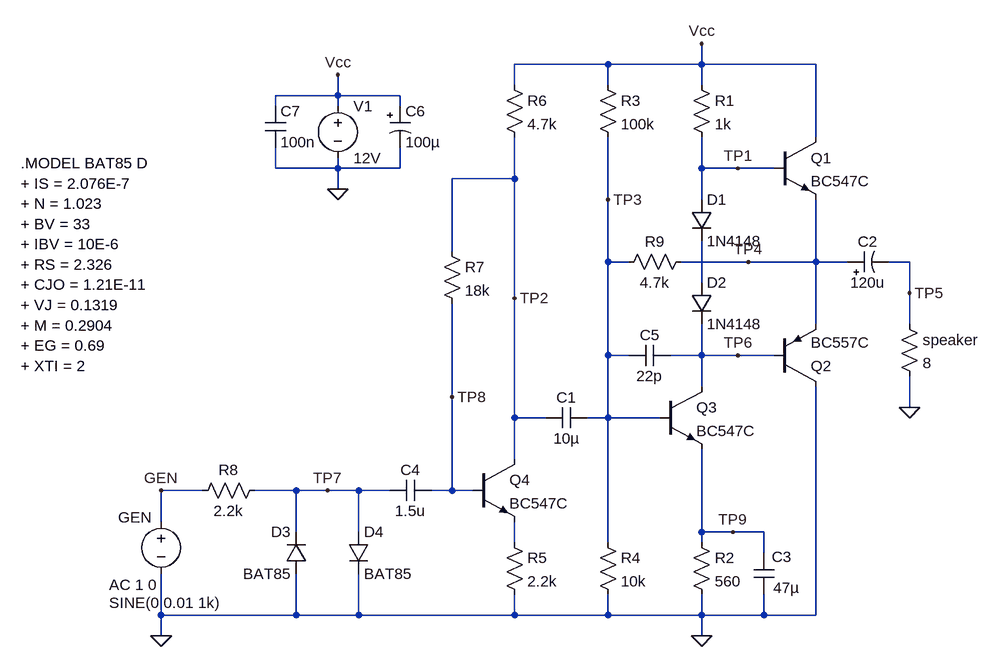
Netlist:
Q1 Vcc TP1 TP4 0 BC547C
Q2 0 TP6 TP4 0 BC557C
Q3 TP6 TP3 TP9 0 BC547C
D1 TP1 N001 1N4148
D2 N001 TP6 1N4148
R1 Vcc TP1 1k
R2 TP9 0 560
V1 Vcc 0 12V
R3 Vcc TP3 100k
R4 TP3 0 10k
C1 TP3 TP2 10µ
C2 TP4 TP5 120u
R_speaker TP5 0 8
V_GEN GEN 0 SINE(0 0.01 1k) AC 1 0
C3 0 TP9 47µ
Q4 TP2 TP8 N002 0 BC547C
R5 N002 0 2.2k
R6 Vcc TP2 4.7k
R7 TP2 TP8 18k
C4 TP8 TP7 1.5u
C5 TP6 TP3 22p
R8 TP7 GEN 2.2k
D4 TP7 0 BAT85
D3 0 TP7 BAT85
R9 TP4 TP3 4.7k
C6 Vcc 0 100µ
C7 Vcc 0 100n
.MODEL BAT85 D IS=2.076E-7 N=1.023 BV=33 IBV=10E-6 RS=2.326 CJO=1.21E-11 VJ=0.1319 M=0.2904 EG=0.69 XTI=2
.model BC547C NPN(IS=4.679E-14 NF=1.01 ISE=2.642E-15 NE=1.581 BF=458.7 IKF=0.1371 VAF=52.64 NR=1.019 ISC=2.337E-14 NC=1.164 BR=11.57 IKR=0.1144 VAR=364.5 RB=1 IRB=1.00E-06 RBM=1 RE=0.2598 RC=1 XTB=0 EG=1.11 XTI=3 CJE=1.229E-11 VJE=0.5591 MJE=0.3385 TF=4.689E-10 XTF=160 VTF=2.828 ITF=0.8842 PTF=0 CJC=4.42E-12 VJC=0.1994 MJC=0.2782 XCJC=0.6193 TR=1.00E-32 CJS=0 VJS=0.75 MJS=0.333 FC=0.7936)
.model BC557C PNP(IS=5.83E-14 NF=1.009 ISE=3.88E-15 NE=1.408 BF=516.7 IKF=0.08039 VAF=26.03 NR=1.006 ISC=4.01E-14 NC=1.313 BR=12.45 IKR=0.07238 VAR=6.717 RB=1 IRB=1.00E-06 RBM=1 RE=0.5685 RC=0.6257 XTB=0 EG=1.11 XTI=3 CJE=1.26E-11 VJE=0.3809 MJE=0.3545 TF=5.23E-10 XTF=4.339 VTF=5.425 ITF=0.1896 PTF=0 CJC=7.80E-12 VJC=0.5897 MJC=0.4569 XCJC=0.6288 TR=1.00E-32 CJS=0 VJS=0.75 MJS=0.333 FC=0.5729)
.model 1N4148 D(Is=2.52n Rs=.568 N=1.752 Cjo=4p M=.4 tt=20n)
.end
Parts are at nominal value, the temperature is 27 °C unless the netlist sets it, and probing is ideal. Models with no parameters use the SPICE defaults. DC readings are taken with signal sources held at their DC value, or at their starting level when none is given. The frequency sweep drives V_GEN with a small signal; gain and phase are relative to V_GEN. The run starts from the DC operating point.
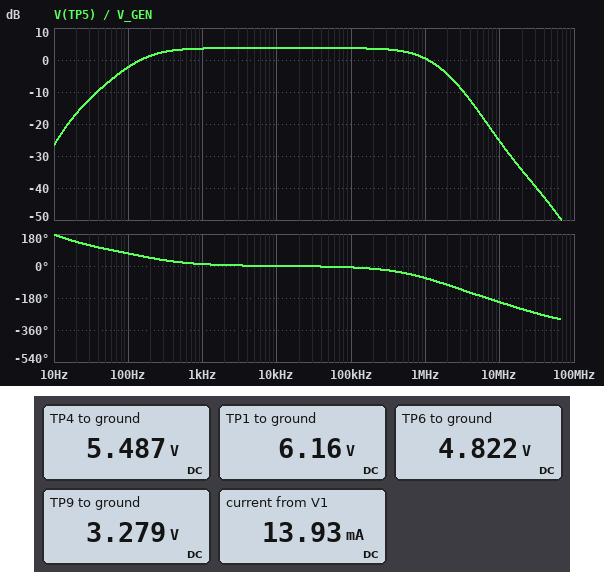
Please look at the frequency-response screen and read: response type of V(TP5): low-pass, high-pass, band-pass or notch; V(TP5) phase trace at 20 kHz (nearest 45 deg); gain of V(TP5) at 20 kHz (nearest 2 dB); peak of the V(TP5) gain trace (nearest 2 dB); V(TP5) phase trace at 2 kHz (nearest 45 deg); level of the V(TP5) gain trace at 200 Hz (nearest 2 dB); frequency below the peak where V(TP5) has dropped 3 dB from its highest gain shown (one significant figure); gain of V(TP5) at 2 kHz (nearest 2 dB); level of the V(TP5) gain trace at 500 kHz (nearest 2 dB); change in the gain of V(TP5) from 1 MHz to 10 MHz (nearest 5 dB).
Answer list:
band-pass
0 deg
4 dB
4 dB
0 deg
2 dB
200 Hz
4 dB
2 dB
-25 dB
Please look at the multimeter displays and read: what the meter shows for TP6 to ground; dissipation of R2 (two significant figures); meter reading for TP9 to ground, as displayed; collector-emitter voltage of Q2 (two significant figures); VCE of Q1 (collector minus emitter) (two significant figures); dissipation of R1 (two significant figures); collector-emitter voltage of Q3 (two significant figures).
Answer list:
4.822 V
19 mW
3.279 V
-5.5 V
6.5 V
34 mW
1.5 V
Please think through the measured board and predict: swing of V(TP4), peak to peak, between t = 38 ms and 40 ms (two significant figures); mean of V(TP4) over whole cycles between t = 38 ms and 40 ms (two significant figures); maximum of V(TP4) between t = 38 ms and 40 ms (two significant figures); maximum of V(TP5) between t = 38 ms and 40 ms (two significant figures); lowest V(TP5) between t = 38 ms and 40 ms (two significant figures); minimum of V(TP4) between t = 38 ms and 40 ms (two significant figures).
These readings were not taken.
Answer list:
31 mV
5.5 V
5.5 V
15 mV
-15 mV
5.5 V
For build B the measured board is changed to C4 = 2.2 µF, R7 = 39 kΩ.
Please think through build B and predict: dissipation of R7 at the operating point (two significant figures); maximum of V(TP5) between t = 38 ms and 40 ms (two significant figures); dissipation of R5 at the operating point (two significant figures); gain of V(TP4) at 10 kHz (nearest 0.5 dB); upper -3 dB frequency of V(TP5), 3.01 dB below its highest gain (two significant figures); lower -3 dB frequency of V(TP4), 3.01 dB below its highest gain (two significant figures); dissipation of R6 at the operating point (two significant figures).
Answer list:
500 nW
17 mV
5.8 mW
5.0 dB
930 kHz
13 Hz
12 mW
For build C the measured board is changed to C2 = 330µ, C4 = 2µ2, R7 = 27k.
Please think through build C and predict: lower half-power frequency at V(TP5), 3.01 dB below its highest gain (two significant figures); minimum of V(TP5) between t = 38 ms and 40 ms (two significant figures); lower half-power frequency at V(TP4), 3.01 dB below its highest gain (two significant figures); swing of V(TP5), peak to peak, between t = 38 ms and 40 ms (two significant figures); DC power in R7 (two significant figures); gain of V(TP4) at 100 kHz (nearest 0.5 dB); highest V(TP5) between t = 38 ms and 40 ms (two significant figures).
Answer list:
68 Hz
-17 mV
15 Hz
33 mV
350 nW
4.5 dB
17 mV
